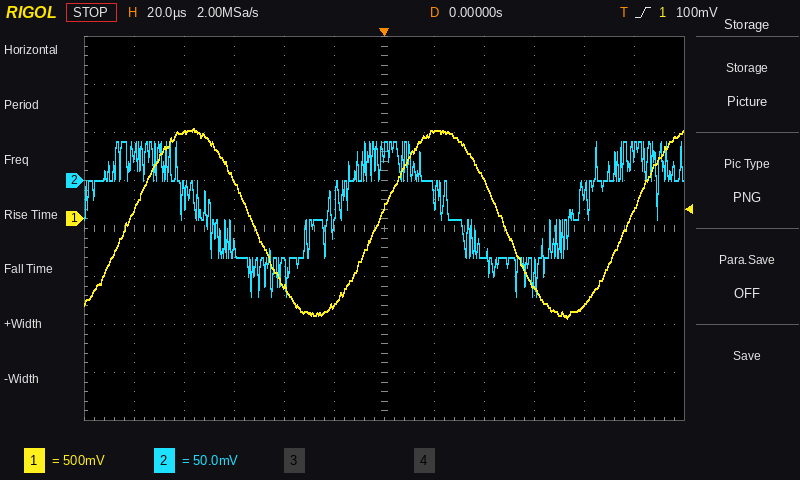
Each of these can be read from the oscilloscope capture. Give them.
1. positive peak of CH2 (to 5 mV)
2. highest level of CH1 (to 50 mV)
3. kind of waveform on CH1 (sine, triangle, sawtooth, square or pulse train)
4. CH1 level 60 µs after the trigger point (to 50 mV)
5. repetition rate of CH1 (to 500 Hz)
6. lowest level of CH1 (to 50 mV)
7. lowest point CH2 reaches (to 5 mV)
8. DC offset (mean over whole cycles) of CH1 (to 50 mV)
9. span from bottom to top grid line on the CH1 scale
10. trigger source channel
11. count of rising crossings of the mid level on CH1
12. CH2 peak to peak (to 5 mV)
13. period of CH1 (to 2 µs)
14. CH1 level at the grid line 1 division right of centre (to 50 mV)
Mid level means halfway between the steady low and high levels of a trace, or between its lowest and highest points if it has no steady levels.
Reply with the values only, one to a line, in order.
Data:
40 mV
950 mV
sine
-700 mV
10.0 kHz
-1.05 V
-120 mV
-50 mV
4 V
CH1
3
160 mV
100 µs
900 mV
